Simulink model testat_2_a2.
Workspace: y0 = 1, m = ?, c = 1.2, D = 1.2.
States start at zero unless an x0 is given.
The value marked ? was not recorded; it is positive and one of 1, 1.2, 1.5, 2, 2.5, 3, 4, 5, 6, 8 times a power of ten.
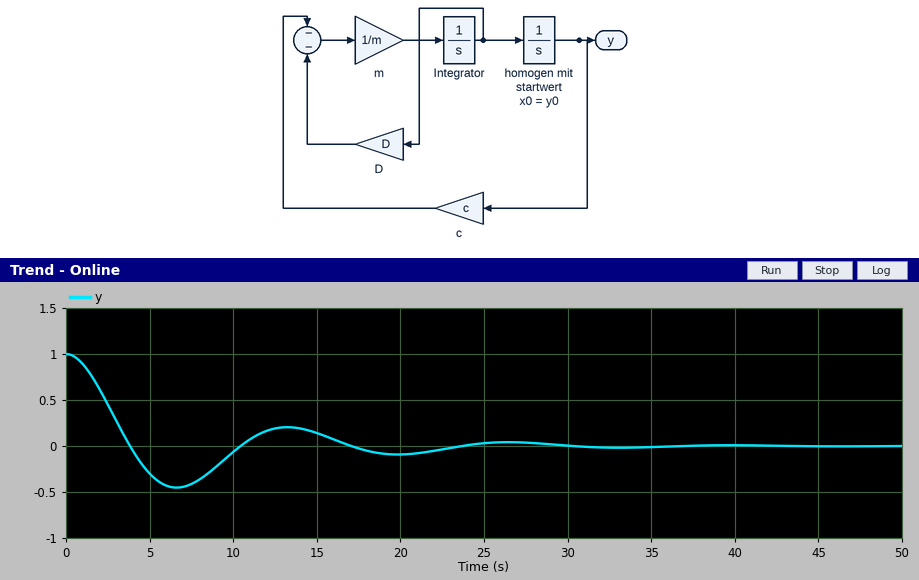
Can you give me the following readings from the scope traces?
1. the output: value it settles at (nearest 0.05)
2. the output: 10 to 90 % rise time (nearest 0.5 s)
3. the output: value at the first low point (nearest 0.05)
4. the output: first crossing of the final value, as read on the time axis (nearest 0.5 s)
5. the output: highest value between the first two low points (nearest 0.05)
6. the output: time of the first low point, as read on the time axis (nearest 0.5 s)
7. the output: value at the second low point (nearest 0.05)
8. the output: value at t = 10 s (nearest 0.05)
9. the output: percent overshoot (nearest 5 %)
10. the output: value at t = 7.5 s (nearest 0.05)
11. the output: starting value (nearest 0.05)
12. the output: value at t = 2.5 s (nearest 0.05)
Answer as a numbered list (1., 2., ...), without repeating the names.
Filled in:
1. 0.00
2. 2.5 s
3. -0.45
4. 4.0 s
5. 0.20
6. 6.5 s
7. -0.10
8. -0.05
9. 45 %
10. -0.40
11. 1.00
12. 0.45
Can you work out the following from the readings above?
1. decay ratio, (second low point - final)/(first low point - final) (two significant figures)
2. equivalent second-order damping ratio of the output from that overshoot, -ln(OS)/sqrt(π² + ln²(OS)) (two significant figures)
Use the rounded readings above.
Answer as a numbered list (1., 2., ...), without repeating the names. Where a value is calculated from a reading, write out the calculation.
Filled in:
1. (-0.1 - 0) / (-0.45 - 0) = 0.22
2. ln(0.45) = -0.799; 0.799 / sqrt(9.870 + 0.638) = 0.25
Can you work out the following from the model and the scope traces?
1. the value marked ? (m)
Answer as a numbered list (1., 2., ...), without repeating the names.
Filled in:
1. 5
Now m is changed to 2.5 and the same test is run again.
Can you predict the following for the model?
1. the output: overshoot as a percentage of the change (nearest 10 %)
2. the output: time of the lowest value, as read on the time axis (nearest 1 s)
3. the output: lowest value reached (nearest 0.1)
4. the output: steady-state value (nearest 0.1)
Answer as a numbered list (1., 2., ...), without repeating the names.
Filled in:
1. 30 %
2. 5 s
3. -0.3
4. 0.0
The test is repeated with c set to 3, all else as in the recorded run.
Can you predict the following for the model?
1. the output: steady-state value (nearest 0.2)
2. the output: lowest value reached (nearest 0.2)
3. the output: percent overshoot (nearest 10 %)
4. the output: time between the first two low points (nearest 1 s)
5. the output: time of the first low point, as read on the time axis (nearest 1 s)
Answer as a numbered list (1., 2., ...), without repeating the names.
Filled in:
1. 0.0
2. -0.6
3. 60 %
4. 8 s
5. 4 s
